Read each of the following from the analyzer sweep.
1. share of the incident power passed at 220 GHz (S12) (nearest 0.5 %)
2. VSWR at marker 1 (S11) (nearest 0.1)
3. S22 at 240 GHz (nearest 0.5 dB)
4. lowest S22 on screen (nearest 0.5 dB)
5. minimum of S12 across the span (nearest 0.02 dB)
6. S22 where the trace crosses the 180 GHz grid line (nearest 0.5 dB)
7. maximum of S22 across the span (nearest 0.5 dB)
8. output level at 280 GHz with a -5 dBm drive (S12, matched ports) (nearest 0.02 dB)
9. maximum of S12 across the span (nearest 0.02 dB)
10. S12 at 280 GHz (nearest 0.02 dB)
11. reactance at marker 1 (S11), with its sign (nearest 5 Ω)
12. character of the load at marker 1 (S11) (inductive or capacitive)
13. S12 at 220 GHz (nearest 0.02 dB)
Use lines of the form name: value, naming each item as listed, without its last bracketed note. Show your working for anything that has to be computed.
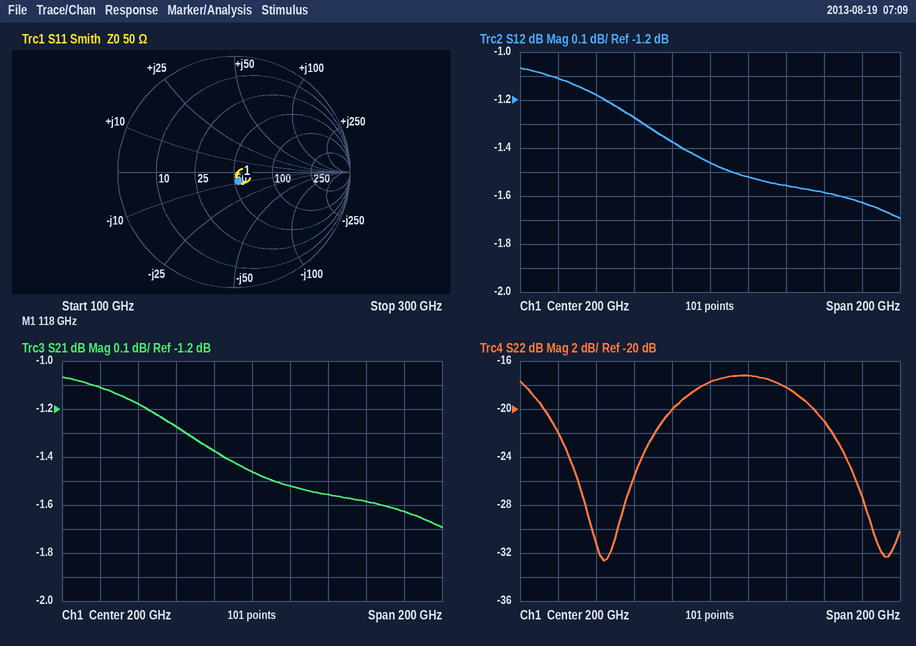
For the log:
share of the incident power passed at 220 GHz (S12): 10^(-1.52/10) ≈ 70.5 %
VSWR at marker 1 (S11): 1.2
S22 at 240 GHz: -18.0 dB
lowest S22 on screen: -32.5 dB
minimum of S12 across the span: -1.70 dB
S22 where the trace crosses the 180 GHz grid line: -20.0 dB
maximum of S22 across the span: -17.0 dB
output level at 280 GHz with a -5 dBm drive (S12, matched ports): -5 dBm + (-1.62 dB) = -6.62 dBm
maximum of S12 across the span: -1.06 dB
S12 at 280 GHz: -1.62 dB
reactance at marker 1 (S11), with its sign: -10 Ω
character of the load at marker 1 (S11): capacitive
S12 at 220 GHz: -1.52 dB
